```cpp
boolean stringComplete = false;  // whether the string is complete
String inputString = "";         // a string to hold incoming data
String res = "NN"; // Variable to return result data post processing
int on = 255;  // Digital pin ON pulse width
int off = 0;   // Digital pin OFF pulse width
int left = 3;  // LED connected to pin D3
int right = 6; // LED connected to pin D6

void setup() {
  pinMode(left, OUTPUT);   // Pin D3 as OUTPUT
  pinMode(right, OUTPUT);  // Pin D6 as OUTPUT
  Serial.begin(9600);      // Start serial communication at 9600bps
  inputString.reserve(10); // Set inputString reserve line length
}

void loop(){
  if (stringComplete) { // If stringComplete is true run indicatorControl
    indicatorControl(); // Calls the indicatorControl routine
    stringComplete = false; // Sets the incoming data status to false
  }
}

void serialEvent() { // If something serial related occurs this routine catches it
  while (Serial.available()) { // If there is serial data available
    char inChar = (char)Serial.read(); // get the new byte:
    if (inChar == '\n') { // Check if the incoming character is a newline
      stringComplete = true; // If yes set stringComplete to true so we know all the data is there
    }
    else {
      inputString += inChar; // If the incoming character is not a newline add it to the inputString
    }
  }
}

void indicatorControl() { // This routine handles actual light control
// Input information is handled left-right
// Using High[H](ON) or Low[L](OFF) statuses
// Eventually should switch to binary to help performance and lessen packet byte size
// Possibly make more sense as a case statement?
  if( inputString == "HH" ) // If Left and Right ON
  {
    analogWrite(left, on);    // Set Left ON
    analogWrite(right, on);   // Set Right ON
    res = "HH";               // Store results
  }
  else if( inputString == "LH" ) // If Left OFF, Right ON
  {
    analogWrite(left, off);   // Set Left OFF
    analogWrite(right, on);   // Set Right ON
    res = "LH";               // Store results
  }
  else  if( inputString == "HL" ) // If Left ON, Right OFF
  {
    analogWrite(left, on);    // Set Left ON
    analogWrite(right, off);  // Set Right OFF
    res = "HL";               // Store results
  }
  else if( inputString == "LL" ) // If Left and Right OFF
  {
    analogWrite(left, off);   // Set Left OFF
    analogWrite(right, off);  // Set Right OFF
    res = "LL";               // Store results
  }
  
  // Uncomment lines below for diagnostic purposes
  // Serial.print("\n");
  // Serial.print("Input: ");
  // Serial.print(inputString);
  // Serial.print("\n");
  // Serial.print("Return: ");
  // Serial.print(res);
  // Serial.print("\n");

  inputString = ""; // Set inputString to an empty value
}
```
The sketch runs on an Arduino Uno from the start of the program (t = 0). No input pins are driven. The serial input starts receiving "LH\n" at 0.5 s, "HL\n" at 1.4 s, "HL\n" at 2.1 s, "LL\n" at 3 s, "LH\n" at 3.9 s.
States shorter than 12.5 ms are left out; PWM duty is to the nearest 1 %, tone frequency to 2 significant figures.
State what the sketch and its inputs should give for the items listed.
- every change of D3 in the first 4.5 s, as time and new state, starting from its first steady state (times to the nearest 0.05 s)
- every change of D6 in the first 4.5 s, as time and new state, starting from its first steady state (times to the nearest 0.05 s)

0 s low; 1.4 s high; 3 s low
0 s low; 0.5 s high; 1.4 s low; 3.9 s high
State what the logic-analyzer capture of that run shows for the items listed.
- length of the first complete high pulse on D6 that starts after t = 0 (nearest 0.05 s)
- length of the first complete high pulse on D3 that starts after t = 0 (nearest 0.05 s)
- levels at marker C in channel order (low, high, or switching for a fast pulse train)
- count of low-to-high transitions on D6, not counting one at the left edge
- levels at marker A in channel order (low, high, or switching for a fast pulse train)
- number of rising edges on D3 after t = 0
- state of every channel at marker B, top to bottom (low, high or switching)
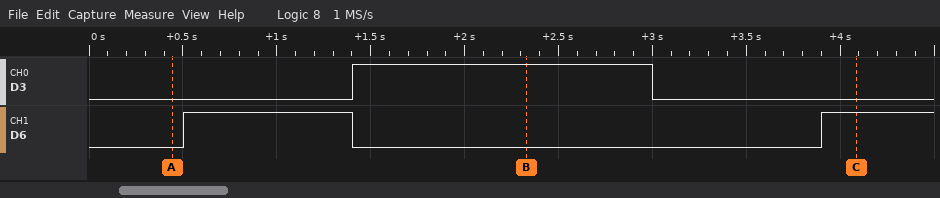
0.90 s
1.60 s
D3 low, D6 high
2
D3 low, D6 low
1
D3 high, D6 low
